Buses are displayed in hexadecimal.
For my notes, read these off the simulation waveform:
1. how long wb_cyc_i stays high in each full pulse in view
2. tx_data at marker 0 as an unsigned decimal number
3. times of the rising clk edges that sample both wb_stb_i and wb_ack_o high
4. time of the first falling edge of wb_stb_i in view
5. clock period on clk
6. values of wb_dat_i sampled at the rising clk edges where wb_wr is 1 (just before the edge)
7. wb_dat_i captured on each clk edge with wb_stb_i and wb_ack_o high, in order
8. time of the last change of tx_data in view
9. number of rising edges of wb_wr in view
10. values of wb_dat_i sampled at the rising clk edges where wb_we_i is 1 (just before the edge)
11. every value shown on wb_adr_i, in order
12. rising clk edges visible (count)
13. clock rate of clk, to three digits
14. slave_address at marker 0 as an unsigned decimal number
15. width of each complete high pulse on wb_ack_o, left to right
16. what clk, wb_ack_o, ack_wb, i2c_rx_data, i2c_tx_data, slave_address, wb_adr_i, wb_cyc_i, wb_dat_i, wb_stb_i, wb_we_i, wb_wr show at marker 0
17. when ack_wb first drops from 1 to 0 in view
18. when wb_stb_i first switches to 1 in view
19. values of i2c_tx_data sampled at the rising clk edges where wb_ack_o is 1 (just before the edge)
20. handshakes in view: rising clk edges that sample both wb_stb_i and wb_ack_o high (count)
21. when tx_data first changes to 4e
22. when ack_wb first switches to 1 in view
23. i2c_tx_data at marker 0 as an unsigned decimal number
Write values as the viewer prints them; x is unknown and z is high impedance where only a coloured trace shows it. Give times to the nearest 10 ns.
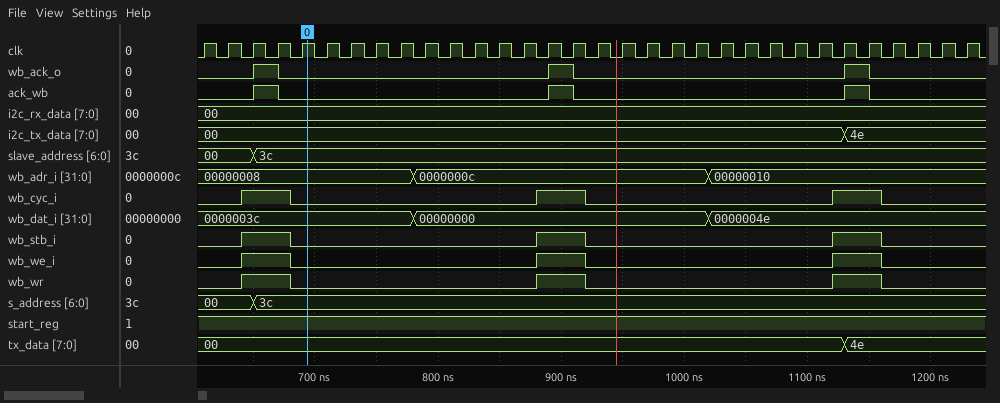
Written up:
40 ns, 40 ns, 40 ns
0
670 ns, 910 ns, 1150 ns
680 ns
20 ns
0000003c, 0000003c, 00000000, 00000000, 0000004e, 0000004e
0000003c, 00000000, 0000004e
1130 ns
3
0000003c, 0000003c, 00000000, 00000000, 0000004e, 0000004e
00000008, 0000000c, 00000010
32
50.0 MHz
60
20 ns, 20 ns, 20 ns
clk=1, wb_ack_o=0, ack_wb=0, i2c_rx_data=00, i2c_tx_data=00, slave_address=3c, wb_adr_i=00000008, wb_cyc_i=0, wb_dat_i=0000003c, wb_stb_i=0, wb_we_i=0, wb_wr=0
670 ns
640 ns
00, 00, 4e
3
1130 ns
650 ns
0
